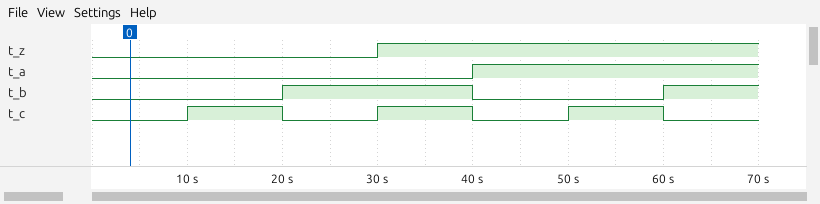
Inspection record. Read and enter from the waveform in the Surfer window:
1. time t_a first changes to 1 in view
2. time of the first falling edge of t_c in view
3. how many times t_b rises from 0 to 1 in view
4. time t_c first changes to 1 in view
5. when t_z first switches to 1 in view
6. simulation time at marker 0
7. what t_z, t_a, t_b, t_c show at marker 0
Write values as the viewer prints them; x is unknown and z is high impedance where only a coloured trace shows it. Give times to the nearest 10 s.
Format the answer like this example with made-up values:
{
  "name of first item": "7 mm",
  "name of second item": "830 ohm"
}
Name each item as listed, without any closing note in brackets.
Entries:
{
  "time t_a first changes to 1 in view": "40 s",
  "time of the first falling edge of t_c in view": "20 s",
  "how many times t_b rises from 0 to 1 in view": "2",
  "time t_c first changes to 1 in view": "10 s",
  "when t_z first switches to 1 in view": "30 s",
  "simulation time at marker 0": "0 s",
  "what t_z, t_a, t_b, t_c show at marker 0": "t_z=0, t_a=0, t_b=0, t_c=0"
}
